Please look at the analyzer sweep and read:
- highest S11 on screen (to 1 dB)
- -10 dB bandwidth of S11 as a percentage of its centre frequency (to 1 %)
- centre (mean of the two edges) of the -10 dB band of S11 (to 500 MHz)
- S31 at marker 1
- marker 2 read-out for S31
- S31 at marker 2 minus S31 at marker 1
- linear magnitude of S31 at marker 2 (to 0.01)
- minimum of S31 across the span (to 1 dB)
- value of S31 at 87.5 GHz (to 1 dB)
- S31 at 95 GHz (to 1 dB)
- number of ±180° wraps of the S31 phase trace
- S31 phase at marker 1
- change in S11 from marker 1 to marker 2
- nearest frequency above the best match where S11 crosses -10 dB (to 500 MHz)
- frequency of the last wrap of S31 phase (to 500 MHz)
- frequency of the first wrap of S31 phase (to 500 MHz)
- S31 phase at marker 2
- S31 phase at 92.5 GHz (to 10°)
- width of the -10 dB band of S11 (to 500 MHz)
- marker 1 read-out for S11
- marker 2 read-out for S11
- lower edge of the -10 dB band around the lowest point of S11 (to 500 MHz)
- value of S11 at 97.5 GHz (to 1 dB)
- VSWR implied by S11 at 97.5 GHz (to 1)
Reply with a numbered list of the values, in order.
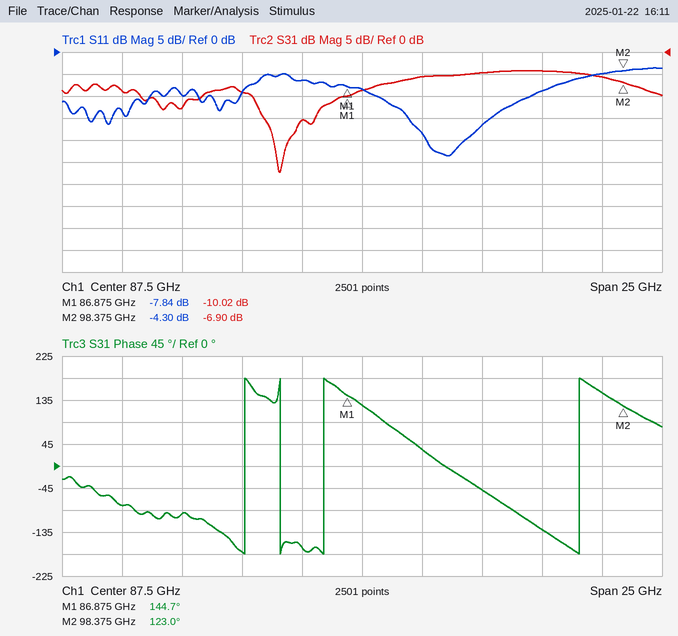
1. -4 dB
2. 7 %
3. 91.5 GHz
4. -10.02 dB
5. -6.90 dB
6. 3.12 dB
7. 0.45
8. -27 dB
9. -9 dB
10. -4 dB
11. 4
12. 144.7°
13. 3.54 dB
14. 94.5 GHz
15. 96.5 GHz
16. 82.5 GHz
17. 123.0°
18. -50°
19. 6.5 GHz
20. -7.84 dB
21. -4.30 dB
22. 88.0 GHz
23. -5 dB
24. 4
